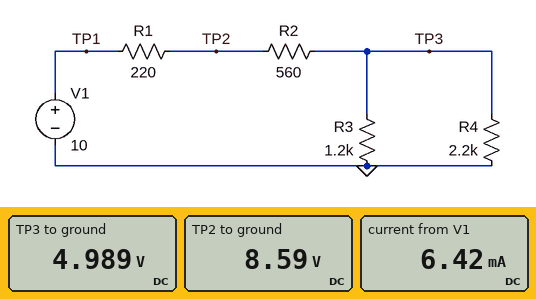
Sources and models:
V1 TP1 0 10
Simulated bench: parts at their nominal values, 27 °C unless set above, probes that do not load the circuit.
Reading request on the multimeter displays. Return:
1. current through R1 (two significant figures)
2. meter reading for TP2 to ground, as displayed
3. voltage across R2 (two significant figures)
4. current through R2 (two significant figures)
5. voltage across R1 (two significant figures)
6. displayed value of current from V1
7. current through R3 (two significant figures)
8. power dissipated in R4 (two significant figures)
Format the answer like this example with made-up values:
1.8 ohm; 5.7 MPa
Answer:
6.4 mA; 8.59 V; 3.6 V; 6.4 mA; 1.4 V; 6.42 mA; 4.2 mA; 11 mW
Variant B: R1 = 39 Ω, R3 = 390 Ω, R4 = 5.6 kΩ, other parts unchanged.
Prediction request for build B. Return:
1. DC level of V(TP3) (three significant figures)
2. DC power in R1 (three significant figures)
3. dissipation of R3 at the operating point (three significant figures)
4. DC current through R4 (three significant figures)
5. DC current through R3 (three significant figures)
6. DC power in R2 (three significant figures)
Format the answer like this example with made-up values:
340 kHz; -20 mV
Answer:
3.78 V; 4.20 mW; 36.7 mW; 676 µA; 9.70 mA; 60.3 mW
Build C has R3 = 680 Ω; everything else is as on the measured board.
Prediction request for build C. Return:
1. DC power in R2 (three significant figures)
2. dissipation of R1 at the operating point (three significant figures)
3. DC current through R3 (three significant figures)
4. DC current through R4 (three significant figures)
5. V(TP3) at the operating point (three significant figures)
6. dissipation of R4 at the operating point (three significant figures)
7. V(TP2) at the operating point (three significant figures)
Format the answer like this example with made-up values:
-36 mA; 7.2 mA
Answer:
33.2 mW; 13.0 mW; 5.88 mA; 1.82 mA; 4.00 V; 7.26 mW; 8.31 V
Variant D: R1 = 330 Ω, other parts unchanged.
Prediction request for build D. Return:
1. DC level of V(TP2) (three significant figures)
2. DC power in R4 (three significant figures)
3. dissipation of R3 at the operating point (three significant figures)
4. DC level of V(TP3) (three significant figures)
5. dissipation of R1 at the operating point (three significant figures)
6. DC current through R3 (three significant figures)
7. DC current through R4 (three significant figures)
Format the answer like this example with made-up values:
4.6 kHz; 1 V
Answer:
8.02 V; 9.87 mW; 18.1 mW; 4.66 V; 11.9 mW; 3.88 mA; 2.12 mA
